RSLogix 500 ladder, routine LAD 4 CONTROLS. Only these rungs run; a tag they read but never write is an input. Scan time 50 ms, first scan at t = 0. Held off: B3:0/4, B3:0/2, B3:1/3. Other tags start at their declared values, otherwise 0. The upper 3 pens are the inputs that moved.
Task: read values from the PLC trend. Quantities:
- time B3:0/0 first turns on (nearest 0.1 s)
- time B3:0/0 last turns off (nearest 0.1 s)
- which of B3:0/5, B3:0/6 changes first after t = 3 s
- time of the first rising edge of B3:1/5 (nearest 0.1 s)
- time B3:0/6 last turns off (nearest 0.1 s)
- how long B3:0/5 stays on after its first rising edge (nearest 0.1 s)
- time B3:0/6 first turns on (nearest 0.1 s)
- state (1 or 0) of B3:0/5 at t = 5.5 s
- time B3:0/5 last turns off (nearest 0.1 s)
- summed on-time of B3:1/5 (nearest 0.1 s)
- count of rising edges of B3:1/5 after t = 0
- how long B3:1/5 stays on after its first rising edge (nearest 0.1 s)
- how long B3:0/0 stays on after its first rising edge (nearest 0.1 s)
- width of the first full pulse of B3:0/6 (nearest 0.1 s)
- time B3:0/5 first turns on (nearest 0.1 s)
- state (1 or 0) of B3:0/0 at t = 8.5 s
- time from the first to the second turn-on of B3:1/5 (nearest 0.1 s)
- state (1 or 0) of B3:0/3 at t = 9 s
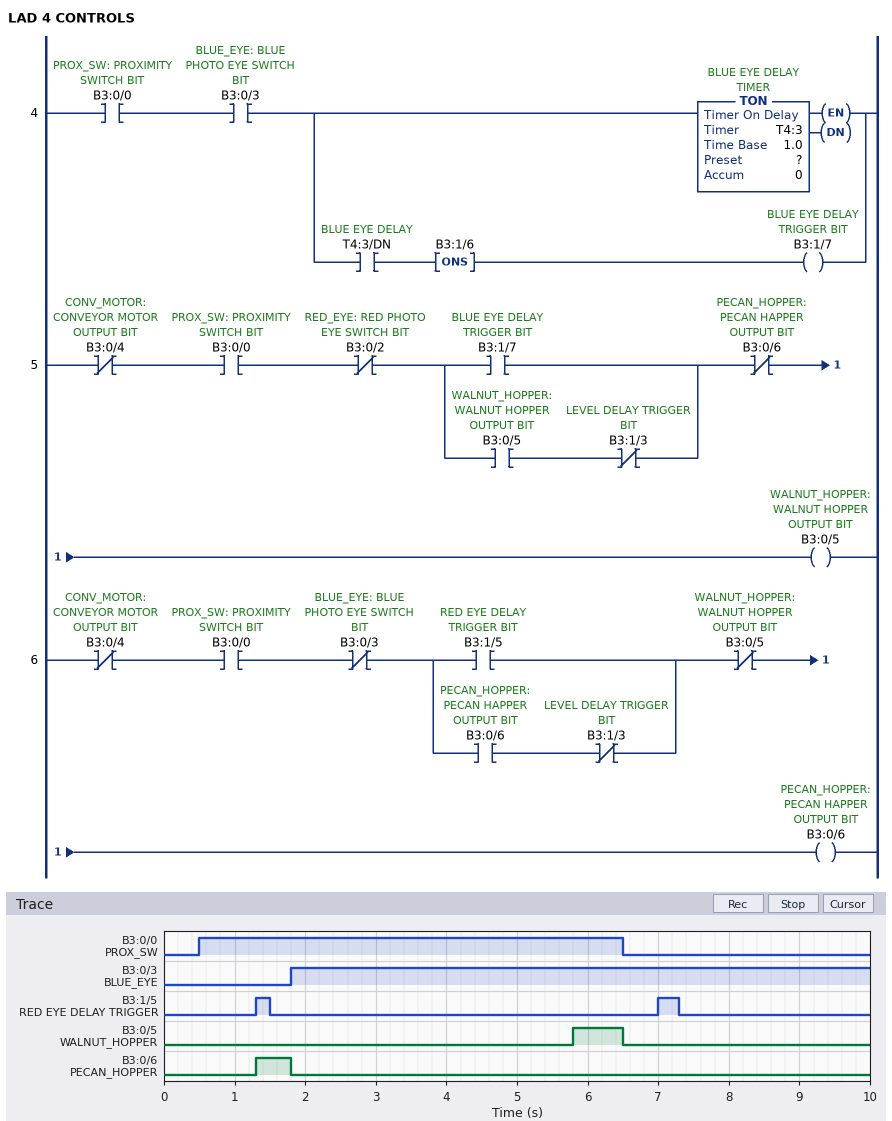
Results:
0.5 s
6.5 s
B3:0/5
1.3 s
1.8 s
0.7 s
1.3 s
0
6.5 s
0.5 s
2
0.2 s
6.0 s
0.5 s
5.8 s
0
5.7 s
1
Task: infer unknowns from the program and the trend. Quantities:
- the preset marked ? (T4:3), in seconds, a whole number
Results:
4 s
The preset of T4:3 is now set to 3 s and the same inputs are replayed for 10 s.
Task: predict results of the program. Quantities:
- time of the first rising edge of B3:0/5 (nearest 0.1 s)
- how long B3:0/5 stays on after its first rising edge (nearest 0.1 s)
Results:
4.8 s
1.7 s
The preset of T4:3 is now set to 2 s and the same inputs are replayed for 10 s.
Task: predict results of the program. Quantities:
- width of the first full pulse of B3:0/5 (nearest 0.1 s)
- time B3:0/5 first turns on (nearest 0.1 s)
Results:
2.7 s
3.8 s
